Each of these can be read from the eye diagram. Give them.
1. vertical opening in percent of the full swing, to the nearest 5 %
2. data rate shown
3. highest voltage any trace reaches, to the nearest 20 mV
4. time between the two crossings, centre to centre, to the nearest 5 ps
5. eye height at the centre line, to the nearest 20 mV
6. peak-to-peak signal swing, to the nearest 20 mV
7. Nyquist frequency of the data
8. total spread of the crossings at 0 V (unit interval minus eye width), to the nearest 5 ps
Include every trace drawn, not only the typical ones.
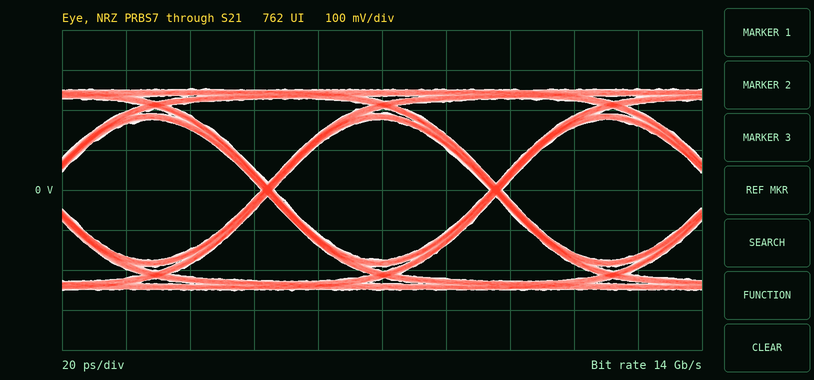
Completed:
70 %
14 Gb/s
260 mV
70 ps
360 mV
500 mV
7 GHz
5 ps
